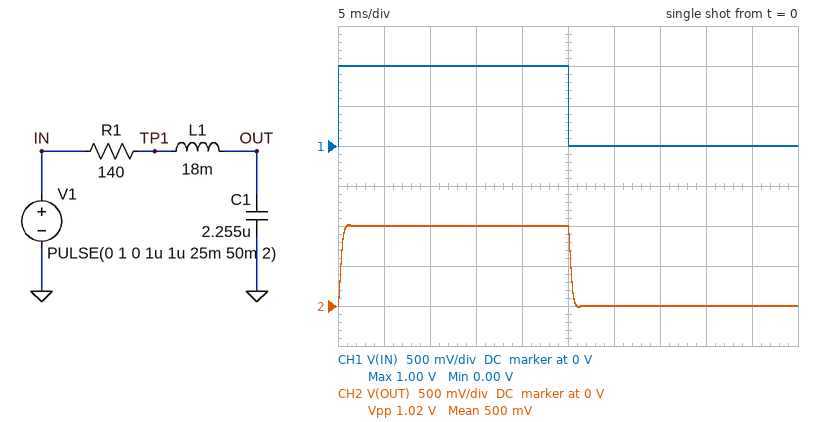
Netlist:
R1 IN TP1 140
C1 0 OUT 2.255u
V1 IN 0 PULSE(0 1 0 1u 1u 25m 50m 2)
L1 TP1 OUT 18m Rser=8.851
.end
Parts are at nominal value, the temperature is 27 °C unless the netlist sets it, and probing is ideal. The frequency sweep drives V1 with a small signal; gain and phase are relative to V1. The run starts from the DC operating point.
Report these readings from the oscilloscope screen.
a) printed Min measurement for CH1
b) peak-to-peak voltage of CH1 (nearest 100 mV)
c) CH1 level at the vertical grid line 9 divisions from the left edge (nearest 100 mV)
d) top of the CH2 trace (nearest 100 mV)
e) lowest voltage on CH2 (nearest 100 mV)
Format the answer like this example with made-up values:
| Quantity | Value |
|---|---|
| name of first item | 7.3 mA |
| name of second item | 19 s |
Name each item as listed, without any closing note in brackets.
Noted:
| Quantity | Value |
|---|---|
| printed Min measurement for CH1 | 0.00 V |
| peak-to-peak voltage of CH1 | 1.0 V |
| CH1 level at the vertical grid line 9 divisions from the left edge | 0 V |
| top of the CH2 trace | 1.0 V |
| lowest voltage on CH2 | 0 V |
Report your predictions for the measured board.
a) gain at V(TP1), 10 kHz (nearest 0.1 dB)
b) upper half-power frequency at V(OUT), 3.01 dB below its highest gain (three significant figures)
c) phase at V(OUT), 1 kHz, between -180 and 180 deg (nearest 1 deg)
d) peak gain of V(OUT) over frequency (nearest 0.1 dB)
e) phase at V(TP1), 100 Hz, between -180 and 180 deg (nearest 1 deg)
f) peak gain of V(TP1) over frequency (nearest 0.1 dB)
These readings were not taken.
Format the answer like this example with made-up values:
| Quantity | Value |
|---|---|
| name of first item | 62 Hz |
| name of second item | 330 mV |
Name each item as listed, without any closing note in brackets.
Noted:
| Quantity | Value |
|---|---|
| gain at V(TP1), 10 kHz | -0.1 dB |
| upper half-power frequency at V(OUT), 3.01 dB below its highest gain | 654 Hz |
| phase at V(OUT), 1 kHz, between -180 and 180 deg | -106 deg |
| peak gain of V(OUT) over frequency | 0 dB |
| phase at V(TP1), 100 Hz, between -180 and 180 deg | -11 deg |
| peak gain of V(TP1) over frequency | 0 dB |
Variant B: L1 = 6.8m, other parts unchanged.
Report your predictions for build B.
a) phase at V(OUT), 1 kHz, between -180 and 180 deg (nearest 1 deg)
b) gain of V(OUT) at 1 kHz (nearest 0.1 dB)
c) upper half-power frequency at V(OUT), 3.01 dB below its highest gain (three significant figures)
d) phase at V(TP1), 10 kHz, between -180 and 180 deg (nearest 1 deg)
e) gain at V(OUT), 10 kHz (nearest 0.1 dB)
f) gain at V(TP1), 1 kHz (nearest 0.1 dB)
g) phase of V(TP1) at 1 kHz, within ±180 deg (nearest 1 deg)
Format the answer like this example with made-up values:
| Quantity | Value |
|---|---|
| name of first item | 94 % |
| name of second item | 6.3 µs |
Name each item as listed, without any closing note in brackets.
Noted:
| Quantity | Value |
|---|---|
| phase at V(OUT), 1 kHz, between -180 and 180 deg | -79 deg |
| gain of V(OUT) at 1 kHz | -6.6 dB |
| upper half-power frequency at V(OUT), 3.01 dB below its highest gain | 547 Hz |
| phase at V(TP1), 10 kHz, between -180 and 180 deg | 18 deg |
| gain at V(OUT), 10 kHz | -36.0 dB |
| gain at V(TP1), 1 kHz | -14.3 dB |
| phase of V(TP1) at 1 kHz, within ±180 deg | -62 deg |
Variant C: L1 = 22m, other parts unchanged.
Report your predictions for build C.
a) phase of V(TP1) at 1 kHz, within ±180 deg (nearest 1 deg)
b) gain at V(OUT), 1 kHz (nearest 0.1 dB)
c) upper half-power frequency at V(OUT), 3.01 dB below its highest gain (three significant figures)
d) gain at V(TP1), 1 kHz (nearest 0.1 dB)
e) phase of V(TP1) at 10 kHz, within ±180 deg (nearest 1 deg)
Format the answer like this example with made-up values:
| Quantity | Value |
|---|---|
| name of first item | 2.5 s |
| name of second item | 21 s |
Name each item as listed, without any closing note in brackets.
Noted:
| Quantity | Value |
|---|---|
| phase of V(TP1) at 1 kHz, within ±180 deg | 58 deg |
| gain at V(OUT), 1 kHz | -7.3 dB |
| upper half-power frequency at V(OUT), 3.01 dB below its highest gain | 668 Hz |
| gain at V(TP1), 1 kHz | -7.6 dB |
| phase of V(TP1) at 10 kHz, within ±180 deg | 6 deg |
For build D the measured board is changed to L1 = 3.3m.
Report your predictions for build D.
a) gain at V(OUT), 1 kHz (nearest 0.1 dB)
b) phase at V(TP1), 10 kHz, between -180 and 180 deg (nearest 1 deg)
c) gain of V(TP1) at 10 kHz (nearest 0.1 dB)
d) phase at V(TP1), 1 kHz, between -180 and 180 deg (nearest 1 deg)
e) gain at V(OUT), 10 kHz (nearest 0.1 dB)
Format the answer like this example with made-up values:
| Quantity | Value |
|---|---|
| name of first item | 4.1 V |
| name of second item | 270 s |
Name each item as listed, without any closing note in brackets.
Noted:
| Quantity | Value |
|---|---|
| gain at V(OUT), 1 kHz | -6.9 dB |
| phase at V(TP1), 10 kHz, between -180 and 180 deg | 34 deg |
| gain of V(TP1) at 10 kHz | -1.9 dB |
| phase at V(TP1), 1 kHz, between -180 and 180 deg | -61 deg |
| gain at V(OUT), 10 kHz | -31.0 dB |
